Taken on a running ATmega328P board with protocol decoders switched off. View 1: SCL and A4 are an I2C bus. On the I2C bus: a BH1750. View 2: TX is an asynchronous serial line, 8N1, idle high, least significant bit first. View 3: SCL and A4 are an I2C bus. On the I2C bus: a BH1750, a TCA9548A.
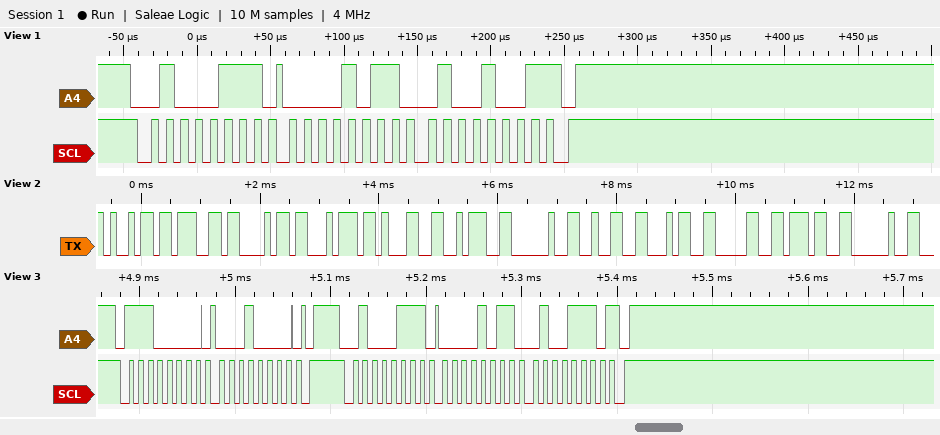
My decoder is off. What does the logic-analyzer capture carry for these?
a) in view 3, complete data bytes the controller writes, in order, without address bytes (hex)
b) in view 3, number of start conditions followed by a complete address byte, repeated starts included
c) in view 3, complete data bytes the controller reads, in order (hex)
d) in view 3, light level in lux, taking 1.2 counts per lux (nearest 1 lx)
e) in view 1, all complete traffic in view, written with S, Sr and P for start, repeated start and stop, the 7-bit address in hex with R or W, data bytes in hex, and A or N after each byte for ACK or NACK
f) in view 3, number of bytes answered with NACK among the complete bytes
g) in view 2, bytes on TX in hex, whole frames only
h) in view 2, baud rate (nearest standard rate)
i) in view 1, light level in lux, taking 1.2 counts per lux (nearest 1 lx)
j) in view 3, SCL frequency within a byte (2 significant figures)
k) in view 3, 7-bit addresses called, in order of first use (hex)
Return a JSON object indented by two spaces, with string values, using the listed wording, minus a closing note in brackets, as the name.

{
  "in view 3, complete data bytes the controller writes, in order, without address bytes": "10",
  "in view 3, number of start conditions followed by a complete address byte, repeated starts included": "2",
  "in view 3, complete data bytes the controller reads, in order": "0B 4E",
  "in view 3, light level in lux, taking 1.2 counts per lux": "2412 lx",
  "in view 1, all complete traffic in view, written with S, Sr and P for start, repeated start and stop, the 7-bit address in hex with R or W, data bytes in hex, and A or N after each byte for ACK or NACK": "S 23R A 0B A 49 N P",
  "in view 3, number of bytes answered with NACK among the complete bytes": "1",
  "in view 2, bytes on TX in hex, whole frames only": "0x69 0x67 0x68 0x74 0x31 0x3A 0x20 0x32 0x34 0x30 0x37 0x20",
  "in view 2, baud rate": "9600 baud",
  "in view 1, light level in lux, taking 1.2 counts per lux": "2408 lx",
  "in view 3, SCL frequency within a byte": "100 kHz",
  "in view 3, 7-bit addresses called, in order of first use": "0x70 0x23"
}
